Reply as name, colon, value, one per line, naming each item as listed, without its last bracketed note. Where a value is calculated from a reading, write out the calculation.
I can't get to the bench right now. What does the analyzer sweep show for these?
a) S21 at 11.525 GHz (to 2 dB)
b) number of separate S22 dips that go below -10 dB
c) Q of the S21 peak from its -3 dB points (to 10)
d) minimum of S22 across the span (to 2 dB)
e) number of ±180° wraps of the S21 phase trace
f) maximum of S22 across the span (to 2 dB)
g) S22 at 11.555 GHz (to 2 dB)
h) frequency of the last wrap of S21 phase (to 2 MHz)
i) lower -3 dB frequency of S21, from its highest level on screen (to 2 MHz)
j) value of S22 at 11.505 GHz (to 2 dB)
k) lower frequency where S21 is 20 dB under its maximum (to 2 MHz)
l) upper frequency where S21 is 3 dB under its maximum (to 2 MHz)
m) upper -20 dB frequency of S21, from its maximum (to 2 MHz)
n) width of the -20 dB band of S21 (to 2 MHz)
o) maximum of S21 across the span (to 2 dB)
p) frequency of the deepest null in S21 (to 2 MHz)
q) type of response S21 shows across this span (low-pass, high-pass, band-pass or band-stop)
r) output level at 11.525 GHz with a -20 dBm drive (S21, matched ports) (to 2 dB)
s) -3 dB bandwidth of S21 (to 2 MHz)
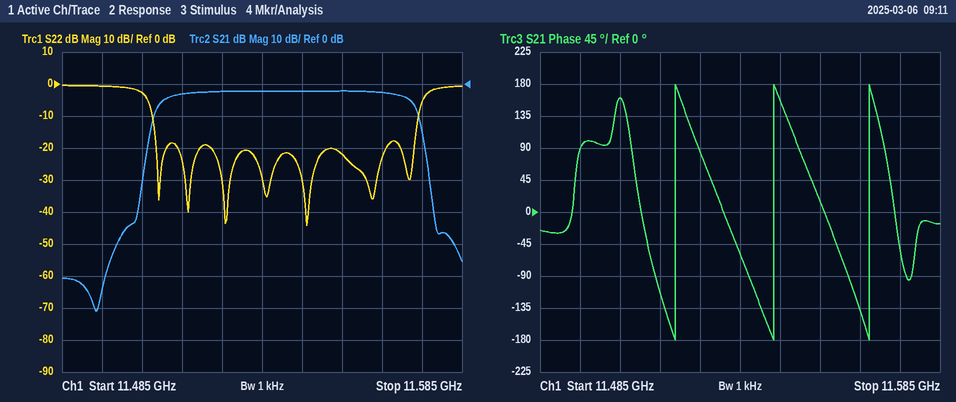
S21 at 11.525 GHz: -2 dB
number of separate S22 dips that go below -10 dB: 7
Q of the S21 peak from its -3 dB points: 11.541 GHz / 62 MHz ≈ 186, so 190 to the nearest 10
minimum of S22 across the span: -44 dB
number of ±180° wraps of the S21 phase trace: 3
maximum of S22 across the span: 0 dB
S22 at 11.555 GHz: -22 dB
frequency of the last wrap of S21 phase: 11.568 GHz
lower -3 dB frequency of S21, from its highest level on screen: 11.510 GHz
value of S22 at 11.505 GHz: -2 dB
lower frequency where S21 is 20 dB under its maximum: 11.506 GHz
upper frequency where S21 is 3 dB under its maximum: 11.572 GHz
upper -20 dB frequency of S21, from its maximum: 11.576 GHz
width of the -20 dB band of S21: 11.576 GHz − 11.506 GHz = 70 MHz
maximum of S21 across the span: -2 dB
frequency of the deepest null in S21: 11.494 GHz
type of response S21 shows across this span: band-pass
output level at 11.525 GHz with a -20 dBm drive (S21, matched ports): -20 dBm + (-2 dB) = -22 dBm
-3 dB bandwidth of S21: 11.572 GHz − 11.510 GHz = 62 MHz
